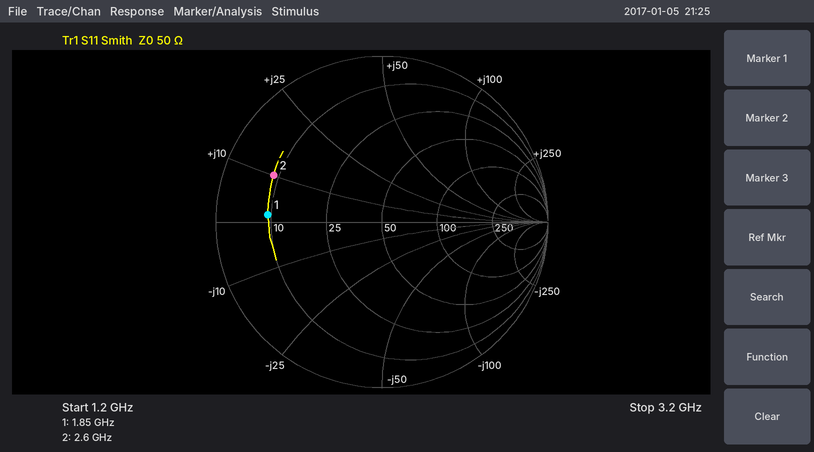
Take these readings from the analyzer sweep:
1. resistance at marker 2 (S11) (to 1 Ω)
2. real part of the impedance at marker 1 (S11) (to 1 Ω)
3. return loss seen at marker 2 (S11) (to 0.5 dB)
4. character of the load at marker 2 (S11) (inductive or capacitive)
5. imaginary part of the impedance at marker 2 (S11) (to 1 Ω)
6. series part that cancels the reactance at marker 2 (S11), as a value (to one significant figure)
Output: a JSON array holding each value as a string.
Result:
["9 Ω", "9 Ω", "3.0 dB", "inductive", "+10 Ω", "6 pF"]
